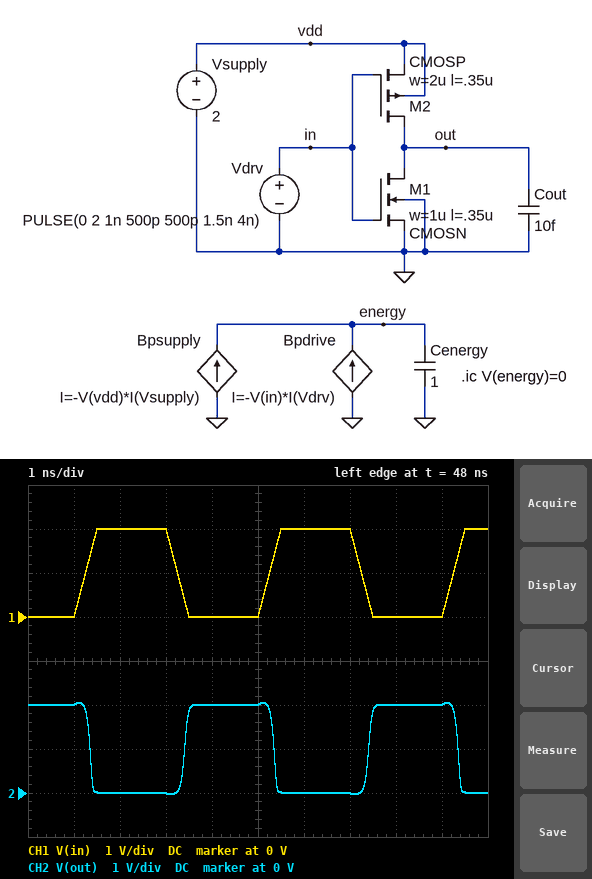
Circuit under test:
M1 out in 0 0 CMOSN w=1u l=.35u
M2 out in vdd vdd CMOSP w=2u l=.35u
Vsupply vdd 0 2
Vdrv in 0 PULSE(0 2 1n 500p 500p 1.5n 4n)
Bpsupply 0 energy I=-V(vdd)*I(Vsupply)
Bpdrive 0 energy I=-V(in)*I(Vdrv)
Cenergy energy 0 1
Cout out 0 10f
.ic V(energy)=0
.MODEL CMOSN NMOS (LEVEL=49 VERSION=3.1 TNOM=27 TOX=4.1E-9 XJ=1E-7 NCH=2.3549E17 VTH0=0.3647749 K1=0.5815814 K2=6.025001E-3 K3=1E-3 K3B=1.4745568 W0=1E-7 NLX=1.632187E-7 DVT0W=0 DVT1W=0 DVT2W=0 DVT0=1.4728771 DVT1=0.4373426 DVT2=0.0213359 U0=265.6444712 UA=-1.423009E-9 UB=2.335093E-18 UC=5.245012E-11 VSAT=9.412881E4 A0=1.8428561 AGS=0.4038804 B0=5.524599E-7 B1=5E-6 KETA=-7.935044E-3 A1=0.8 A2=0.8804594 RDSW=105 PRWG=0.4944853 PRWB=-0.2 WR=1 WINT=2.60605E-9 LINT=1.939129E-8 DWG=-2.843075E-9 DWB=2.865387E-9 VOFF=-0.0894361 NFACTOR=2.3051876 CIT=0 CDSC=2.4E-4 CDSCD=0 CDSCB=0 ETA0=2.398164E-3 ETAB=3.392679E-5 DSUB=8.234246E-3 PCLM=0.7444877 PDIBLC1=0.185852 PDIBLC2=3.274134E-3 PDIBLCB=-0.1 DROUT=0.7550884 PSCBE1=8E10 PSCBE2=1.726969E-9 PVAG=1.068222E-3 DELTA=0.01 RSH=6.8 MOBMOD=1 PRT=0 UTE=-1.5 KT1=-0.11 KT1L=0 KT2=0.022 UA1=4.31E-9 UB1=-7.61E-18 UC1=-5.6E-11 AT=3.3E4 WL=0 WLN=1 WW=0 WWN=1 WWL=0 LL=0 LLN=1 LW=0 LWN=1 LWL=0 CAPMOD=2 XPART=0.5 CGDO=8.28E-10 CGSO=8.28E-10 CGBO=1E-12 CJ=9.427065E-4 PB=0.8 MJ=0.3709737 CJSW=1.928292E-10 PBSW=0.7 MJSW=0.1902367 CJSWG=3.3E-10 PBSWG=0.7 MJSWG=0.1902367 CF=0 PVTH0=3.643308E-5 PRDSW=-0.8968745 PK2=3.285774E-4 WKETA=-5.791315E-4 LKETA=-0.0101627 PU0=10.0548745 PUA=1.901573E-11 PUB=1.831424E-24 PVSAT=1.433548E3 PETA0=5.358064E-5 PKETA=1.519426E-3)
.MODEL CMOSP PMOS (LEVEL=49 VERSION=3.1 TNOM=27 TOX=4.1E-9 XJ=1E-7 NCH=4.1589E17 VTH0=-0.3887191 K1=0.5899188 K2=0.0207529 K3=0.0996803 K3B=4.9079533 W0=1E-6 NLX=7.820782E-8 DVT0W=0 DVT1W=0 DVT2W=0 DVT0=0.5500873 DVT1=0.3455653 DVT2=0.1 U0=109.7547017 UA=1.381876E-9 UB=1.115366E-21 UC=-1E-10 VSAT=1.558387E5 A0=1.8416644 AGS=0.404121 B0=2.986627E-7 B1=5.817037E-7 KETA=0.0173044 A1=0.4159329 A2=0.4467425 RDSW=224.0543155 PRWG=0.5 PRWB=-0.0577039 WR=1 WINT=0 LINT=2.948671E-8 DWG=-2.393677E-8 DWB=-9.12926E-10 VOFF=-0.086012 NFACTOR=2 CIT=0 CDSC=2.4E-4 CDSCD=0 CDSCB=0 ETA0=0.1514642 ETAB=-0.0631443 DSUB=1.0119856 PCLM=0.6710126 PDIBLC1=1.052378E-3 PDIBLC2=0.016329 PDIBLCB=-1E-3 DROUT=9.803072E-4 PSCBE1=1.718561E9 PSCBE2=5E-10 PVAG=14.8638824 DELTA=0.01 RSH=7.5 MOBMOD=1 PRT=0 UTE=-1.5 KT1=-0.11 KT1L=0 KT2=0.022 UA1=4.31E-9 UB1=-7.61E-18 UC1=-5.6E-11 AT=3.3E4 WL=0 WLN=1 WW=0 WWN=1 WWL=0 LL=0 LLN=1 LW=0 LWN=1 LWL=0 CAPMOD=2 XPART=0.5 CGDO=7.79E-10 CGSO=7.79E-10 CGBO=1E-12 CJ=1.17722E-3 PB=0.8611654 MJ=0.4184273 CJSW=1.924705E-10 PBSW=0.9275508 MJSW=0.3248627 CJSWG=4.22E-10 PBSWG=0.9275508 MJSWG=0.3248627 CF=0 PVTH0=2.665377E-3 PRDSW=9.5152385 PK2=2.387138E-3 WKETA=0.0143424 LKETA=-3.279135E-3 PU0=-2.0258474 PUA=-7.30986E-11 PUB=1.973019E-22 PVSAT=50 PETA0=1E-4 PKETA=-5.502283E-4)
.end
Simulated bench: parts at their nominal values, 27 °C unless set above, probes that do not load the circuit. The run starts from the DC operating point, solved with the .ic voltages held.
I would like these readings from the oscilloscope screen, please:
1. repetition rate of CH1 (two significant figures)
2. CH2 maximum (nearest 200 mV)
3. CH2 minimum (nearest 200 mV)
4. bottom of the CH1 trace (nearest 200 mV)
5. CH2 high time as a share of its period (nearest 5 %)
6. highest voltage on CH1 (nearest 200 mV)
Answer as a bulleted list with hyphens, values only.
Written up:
- 250 MHz
- 2.0 V
- 0 V
- 0 V
- 50 %
- 2.0 V
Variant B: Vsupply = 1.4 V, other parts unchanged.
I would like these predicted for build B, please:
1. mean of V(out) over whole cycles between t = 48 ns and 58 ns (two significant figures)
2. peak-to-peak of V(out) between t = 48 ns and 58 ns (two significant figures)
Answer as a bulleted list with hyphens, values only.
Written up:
- 630 mV
- 1.5 V
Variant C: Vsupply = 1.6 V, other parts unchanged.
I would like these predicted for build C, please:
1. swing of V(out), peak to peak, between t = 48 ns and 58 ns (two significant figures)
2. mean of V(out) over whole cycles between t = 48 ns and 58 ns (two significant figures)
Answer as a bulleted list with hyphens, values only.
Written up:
- 1.7 V
- 740 mV
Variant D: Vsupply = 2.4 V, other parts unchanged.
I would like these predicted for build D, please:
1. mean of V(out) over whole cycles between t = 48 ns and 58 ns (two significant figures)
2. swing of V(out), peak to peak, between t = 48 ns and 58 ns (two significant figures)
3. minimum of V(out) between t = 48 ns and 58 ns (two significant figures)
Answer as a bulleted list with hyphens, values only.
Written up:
- 1.2 V
- 2.5 V
- -18 mV
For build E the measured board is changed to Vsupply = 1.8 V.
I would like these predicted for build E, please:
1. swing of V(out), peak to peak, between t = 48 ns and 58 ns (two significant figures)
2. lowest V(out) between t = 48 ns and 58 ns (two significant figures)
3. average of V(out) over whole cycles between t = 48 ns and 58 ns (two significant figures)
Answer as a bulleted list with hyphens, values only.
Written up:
- 1.9 V
- -26 mV
- 850 mV
